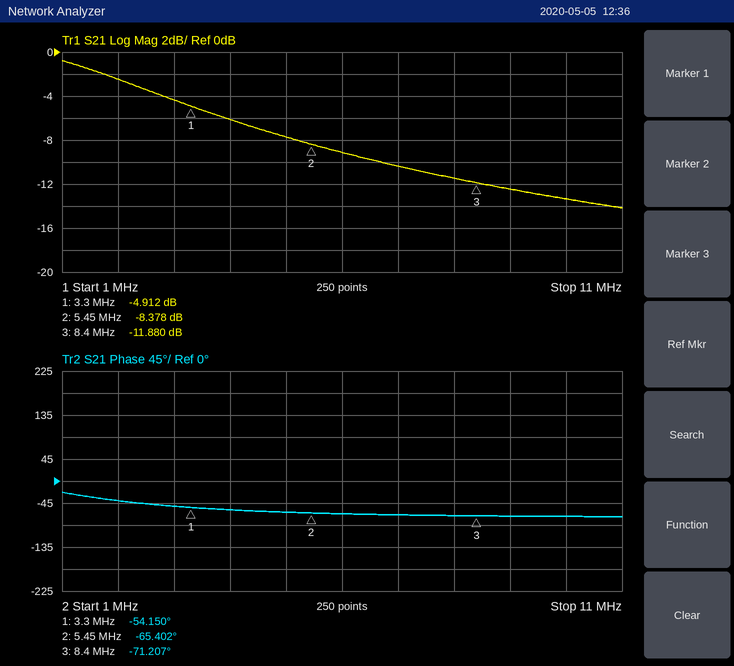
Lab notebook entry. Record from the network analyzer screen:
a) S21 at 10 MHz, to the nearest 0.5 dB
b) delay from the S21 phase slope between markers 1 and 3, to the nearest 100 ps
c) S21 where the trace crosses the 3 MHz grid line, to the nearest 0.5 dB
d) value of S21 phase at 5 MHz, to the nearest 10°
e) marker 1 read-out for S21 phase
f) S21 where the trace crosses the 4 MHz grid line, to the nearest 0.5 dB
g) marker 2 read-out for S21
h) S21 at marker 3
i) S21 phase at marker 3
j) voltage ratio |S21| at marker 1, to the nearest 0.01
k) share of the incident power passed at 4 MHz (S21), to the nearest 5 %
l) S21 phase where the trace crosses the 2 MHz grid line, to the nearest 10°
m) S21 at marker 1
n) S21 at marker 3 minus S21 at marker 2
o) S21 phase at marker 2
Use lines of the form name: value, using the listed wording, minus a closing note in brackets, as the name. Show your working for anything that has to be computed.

S21 at 10 MHz, to the nearest 0.5 dB: -13.5 dB
delay from the S21 phase slope between markers 1 and 3, to the nearest 100 ps: −(-71.207° − (-54.15°))/(360° × 5.1 MHz) ≈ 9.3 ns
S21 where the trace crosses the 3 MHz grid line, to the nearest 0.5 dB: -4.5 dB
value of S21 phase at 5 MHz, to the nearest 10°: -60°
marker 1 read-out for S21 phase: -54.150°
S21 where the trace crosses the 4 MHz grid line, to the nearest 0.5 dB: -6.0 dB
marker 2 read-out for S21: -8.378 dB
S21 at marker 3: -11.880 dB
S21 phase at marker 3: -71.207°
voltage ratio |S21| at marker 1, to the nearest 0.01: 10^(-4.912/20) ≈ 0.57
share of the incident power passed at 4 MHz (S21), to the nearest 5 %: 10^(-6/10) ≈ 25 %
S21 phase where the trace crosses the 2 MHz grid line, to the nearest 10°: -40°
S21 at marker 1: -4.912 dB
S21 at marker 3 minus S21 at marker 2: -11.88 − (-8.378) = -3.502 dB
S21 phase at marker 2: -65.402°
